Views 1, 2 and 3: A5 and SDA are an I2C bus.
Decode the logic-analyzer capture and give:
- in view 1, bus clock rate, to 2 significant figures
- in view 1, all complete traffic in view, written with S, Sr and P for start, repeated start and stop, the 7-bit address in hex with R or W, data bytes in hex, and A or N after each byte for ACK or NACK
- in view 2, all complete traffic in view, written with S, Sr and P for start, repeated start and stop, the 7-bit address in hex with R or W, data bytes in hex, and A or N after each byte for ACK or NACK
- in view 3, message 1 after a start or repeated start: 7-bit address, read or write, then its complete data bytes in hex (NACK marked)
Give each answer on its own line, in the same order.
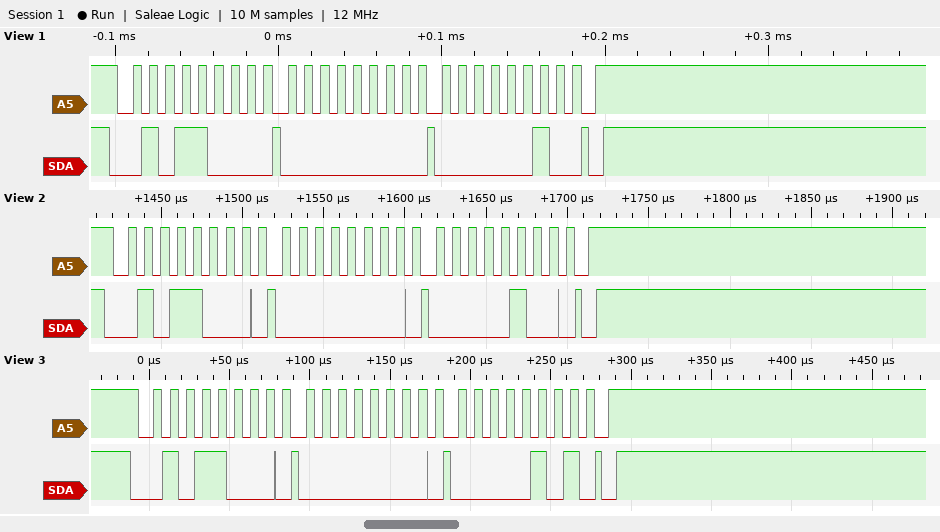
100 kHz
S 2CW A 00 A 02 A P
S 2CW A 00 A 04 A P
0x2C write: 00 05
